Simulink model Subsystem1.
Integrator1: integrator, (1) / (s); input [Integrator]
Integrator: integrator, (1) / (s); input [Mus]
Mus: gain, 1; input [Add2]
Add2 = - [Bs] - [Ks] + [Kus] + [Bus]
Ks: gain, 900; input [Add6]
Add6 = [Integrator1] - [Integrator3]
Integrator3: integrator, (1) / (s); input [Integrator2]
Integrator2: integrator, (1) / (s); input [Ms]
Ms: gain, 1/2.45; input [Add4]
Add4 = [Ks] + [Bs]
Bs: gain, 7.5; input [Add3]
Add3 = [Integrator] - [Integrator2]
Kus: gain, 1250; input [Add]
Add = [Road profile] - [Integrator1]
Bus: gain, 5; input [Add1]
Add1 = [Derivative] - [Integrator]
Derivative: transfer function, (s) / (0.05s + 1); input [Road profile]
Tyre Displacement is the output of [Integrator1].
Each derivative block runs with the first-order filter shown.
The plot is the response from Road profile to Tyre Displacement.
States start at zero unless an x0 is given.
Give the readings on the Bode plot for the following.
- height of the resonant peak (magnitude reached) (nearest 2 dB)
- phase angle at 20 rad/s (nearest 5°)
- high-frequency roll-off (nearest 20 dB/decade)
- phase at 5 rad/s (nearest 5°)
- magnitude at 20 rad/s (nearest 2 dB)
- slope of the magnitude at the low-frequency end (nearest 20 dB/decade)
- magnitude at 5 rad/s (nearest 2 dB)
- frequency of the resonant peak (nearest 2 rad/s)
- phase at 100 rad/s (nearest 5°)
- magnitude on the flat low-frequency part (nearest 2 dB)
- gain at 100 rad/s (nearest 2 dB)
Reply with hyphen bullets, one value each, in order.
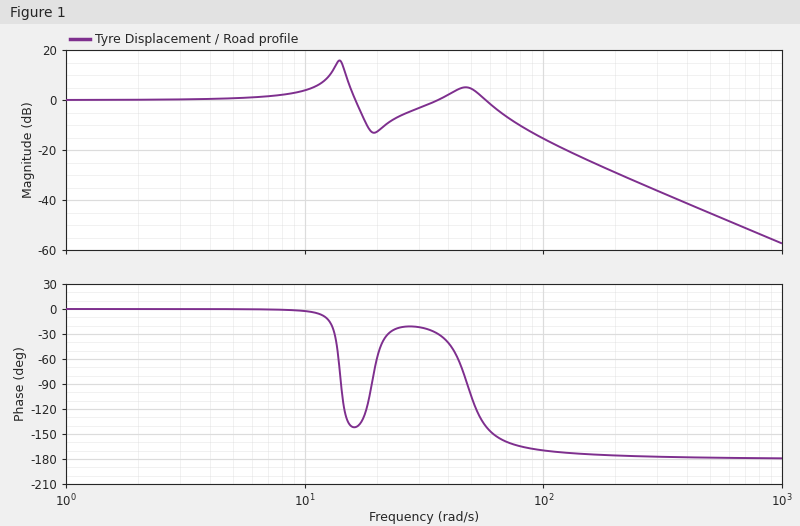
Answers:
- 16 dB
- -60°
- -40 dB/decade
- 0°
- -12 dB
- 0 dB/decade
- 0 dB
- 14 rad/s
- -170°
- 0 dB
- -16 dB
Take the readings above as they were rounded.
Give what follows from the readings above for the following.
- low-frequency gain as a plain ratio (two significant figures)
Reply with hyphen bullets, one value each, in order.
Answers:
- 1.0
